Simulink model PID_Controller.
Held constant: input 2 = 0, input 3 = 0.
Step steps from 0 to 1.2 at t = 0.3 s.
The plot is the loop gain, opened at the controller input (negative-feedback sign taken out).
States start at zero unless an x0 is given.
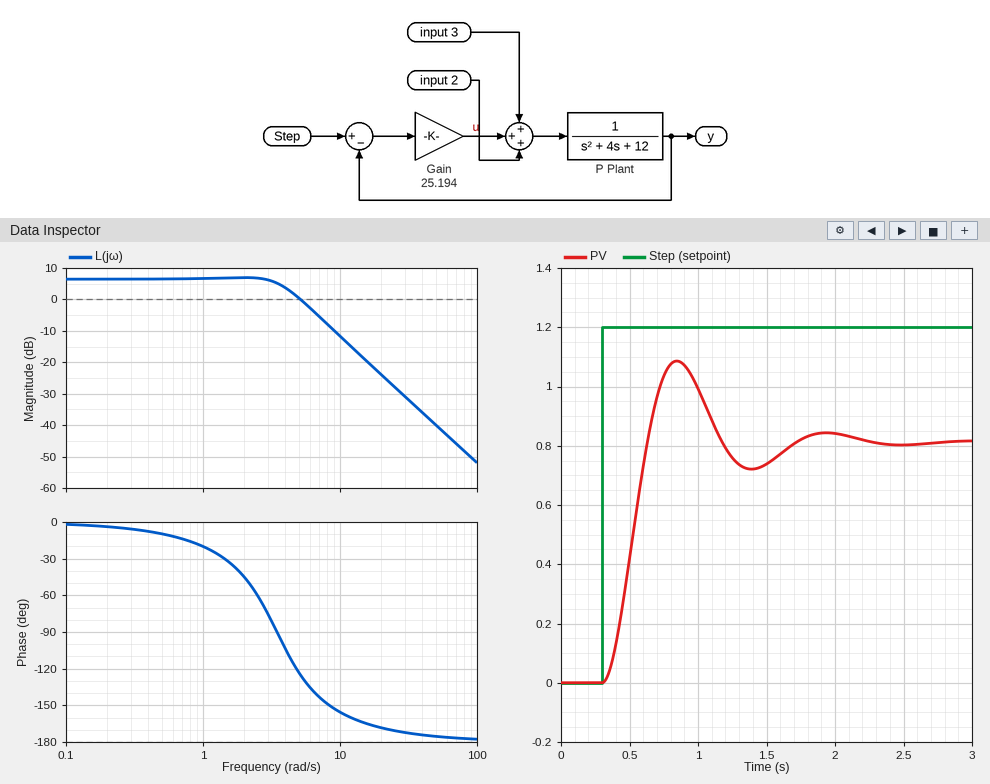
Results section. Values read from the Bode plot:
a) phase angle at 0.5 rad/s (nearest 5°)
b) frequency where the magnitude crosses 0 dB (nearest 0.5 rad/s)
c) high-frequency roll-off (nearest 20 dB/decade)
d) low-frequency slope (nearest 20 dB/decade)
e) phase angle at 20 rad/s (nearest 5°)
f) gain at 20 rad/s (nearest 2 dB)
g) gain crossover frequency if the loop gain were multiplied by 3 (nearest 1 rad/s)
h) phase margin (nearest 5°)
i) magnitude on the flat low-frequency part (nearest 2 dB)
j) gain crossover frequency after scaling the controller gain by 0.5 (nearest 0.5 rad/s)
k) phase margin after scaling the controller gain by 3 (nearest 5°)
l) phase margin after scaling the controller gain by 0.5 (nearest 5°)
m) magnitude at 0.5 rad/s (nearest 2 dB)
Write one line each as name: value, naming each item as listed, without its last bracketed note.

phase angle at 0.5 rad/s: -10°
frequency where the magnitude crosses 0 dB: 5.0 rad/s
high-frequency roll-off: -40 dB/decade
low-frequency slope: 0 dB/decade
phase angle at 20 rad/s: -170°
gain at 20 rad/s: -24 dB
gain crossover frequency if the loop gain were multiplied by 3: 9 rad/s
phase margin: 55°
magnitude on the flat low-frequency part: 6 dB
gain crossover frequency after scaling the controller gain by 0.5: 3.0 rad/s
phase margin after scaling the controller gain by 3: 30°
phase margin after scaling the controller gain by 0.5: 100°
magnitude at 0.5 rad/s: 6 dB
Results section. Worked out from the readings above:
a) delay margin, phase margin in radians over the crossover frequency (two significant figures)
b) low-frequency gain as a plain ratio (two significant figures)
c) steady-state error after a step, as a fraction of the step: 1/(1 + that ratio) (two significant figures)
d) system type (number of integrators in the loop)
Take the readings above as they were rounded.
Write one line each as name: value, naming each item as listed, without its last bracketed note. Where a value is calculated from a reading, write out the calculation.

delay margin, phase margin in radians over the crossover frequency: 55 × π / 180 / 5 = 0.19 s
low-frequency gain as a plain ratio: 10^(6 / 20) = 2.0
steady-state error after a step, as a fraction of the step: 1/(1 + that ratio): 1 / (1 + 2) = 0.33
system type: 0
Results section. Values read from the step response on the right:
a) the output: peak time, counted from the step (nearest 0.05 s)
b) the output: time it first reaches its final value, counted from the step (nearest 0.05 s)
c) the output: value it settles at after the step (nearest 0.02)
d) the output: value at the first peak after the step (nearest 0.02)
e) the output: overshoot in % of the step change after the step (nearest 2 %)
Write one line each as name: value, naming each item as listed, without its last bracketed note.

the output: peak time, counted from the step: 0.55 s
the output: time it first reaches its final value, counted from the step: 0.35 s
the output: value it settles at after the step: 0.82
the output: value at the first peak after the step: 1.08
the output: overshoot in % of the step change after the step: 34 %
